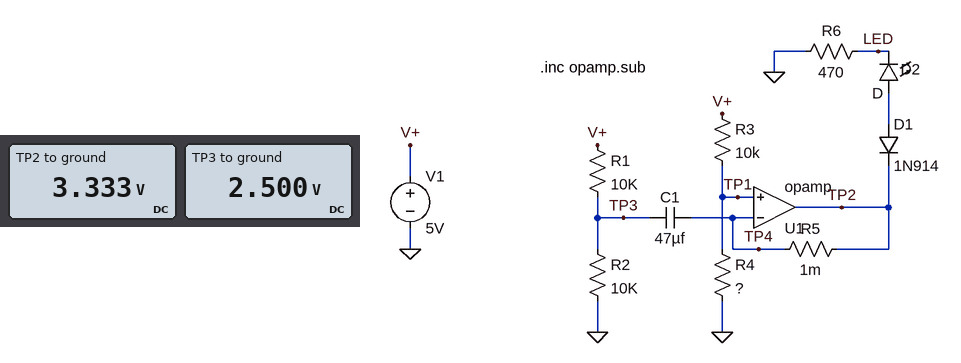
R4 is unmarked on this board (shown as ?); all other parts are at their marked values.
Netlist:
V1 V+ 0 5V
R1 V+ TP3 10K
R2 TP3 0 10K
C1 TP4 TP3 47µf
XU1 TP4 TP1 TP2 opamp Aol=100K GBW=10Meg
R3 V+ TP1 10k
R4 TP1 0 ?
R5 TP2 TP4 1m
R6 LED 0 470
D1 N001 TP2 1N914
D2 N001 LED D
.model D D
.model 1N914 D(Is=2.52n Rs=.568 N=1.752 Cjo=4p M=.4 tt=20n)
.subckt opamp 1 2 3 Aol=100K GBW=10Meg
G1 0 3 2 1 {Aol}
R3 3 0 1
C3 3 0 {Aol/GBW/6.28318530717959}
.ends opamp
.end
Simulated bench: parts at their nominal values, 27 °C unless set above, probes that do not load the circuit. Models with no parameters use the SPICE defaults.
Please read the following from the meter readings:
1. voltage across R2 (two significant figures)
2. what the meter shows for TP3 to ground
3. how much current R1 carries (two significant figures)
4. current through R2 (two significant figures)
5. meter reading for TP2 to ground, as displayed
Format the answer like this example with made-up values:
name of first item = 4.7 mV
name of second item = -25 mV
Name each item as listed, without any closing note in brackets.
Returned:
voltage across R2 = 2.5 V
what the meter shows for TP3 to ground = 2.500 V
how much current R1 carries = 250 µA
current through R2 = 250 µA
meter reading for TP2 to ground, as displayed = 3.333 V
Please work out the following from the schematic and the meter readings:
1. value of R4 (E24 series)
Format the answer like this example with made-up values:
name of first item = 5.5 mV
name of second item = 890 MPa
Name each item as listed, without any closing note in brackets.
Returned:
value of R4 = 20 kΩ
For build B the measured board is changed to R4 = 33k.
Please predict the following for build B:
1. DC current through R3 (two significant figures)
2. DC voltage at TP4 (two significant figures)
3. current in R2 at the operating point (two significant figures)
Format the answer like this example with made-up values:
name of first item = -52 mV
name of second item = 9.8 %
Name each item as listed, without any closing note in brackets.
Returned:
DC current through R3 = 120 µA
DC voltage at TP4 = 3.8 V
current in R2 at the operating point = 250 µA
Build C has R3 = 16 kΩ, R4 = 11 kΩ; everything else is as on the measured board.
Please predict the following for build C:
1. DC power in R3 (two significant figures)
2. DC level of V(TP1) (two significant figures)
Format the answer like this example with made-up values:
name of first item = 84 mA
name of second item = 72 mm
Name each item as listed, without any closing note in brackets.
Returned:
DC power in R3 = 550 µW
DC level of V(TP1) = 2.0 V
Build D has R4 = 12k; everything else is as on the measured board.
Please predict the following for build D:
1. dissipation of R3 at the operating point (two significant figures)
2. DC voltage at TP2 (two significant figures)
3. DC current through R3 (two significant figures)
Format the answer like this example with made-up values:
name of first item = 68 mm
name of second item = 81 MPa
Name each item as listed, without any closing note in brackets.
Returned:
dissipation of R3 at the operating point = 520 µW
DC voltage at TP2 = 2.7 V
DC current through R3 = 230 µA
